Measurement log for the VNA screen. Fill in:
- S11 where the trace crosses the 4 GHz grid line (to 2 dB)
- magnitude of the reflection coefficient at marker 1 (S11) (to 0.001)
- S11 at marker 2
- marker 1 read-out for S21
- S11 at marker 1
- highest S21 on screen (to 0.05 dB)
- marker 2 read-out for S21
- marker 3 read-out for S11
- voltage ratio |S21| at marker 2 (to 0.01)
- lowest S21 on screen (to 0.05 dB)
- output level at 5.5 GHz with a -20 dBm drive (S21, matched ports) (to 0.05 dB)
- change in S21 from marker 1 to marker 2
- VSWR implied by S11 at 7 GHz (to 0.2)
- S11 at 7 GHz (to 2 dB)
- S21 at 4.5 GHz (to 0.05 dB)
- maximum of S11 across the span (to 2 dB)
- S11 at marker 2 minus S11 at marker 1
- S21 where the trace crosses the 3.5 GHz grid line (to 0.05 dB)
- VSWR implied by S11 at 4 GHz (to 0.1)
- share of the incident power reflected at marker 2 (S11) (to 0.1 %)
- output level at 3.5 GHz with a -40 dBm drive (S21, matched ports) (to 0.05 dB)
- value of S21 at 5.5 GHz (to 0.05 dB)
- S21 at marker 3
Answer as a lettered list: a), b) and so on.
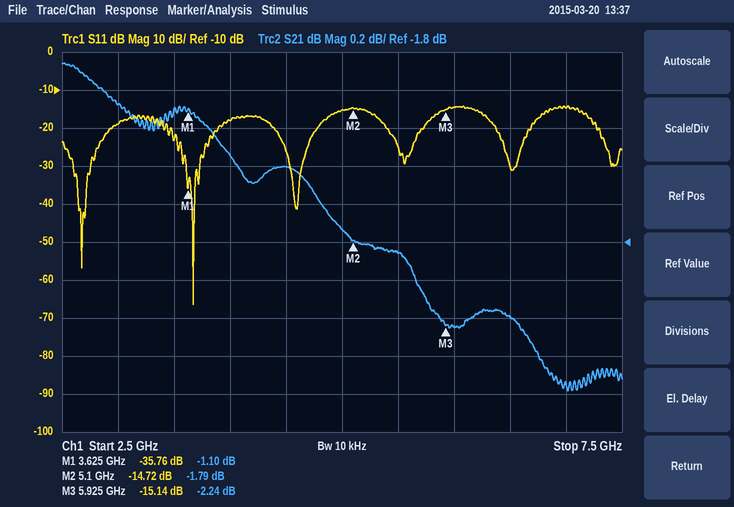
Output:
a) -18 dB
b) 0.016
c) -14.72 dB
d) -1.10 dB
e) -35.76 dB
f) -0.85 dB
g) -1.79 dB
h) -15.14 dB
i) 0.81
j) -2.60 dB
k) -21.85 dBm
l) -0.69 dB
m) 1.4
n) -14 dB
o) -1.40 dB
p) -14 dB
q) 21.04 dB
r) -1.10 dB
s) 1.3
t) 3.4 %
u) -41.10 dBm
v) -1.85 dB
w) -2.24 dB
